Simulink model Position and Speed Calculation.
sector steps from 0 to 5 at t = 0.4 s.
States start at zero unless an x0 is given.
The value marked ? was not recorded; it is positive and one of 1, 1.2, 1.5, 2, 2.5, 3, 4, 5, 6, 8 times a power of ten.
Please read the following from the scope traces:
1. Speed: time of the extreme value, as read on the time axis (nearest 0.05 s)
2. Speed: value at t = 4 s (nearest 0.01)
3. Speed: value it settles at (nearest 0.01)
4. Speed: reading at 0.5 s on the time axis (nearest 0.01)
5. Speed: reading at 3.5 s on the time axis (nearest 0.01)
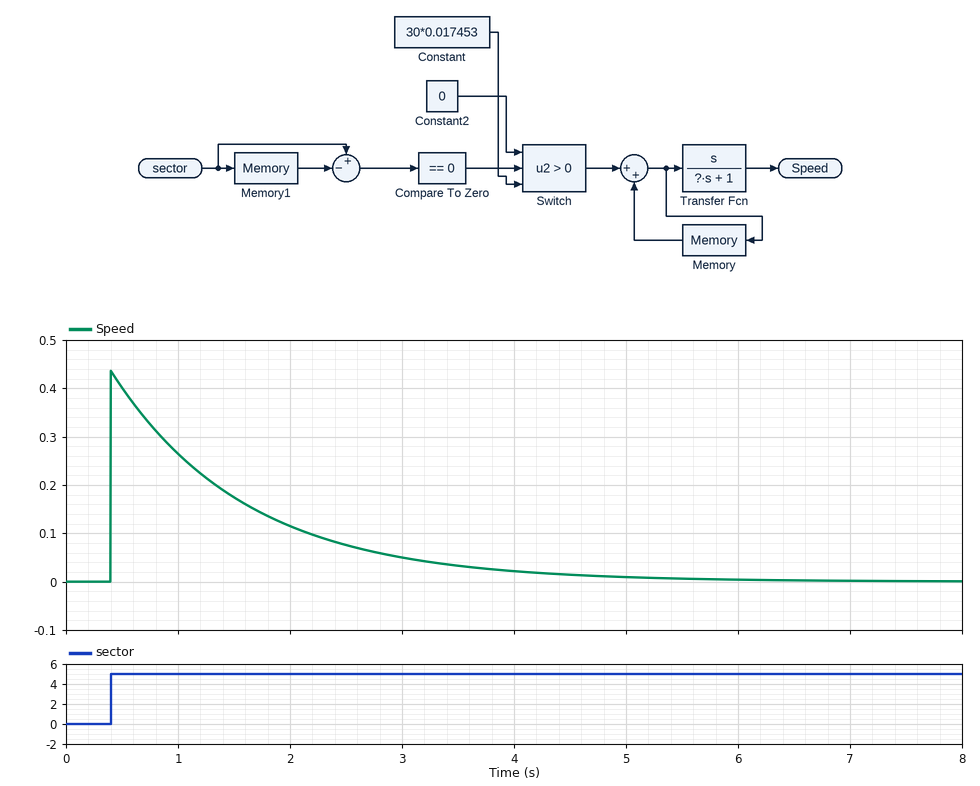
0.40 s
0.02
0.00
0.40
0.03
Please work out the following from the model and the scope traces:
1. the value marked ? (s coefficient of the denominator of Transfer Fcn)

1.2
